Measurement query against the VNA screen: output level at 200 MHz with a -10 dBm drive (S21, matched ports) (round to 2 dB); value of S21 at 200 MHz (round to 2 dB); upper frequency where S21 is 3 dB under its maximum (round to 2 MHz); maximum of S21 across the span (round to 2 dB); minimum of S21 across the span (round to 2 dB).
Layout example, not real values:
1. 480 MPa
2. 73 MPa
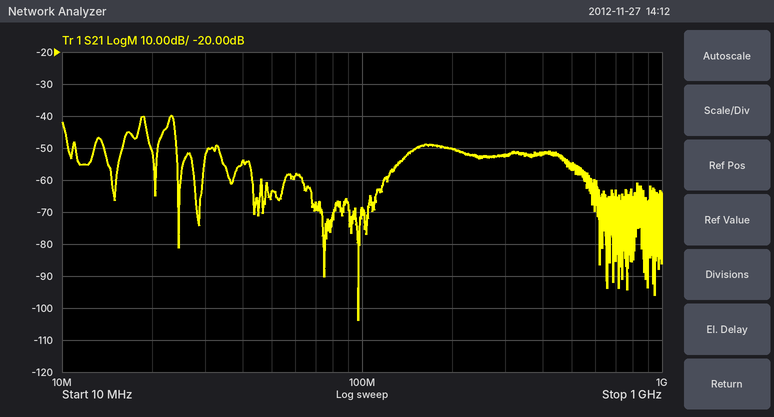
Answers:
1. -60 dBm
2. -50 dB
3. 24 MHz
4. -40 dB
5. -104 dB
